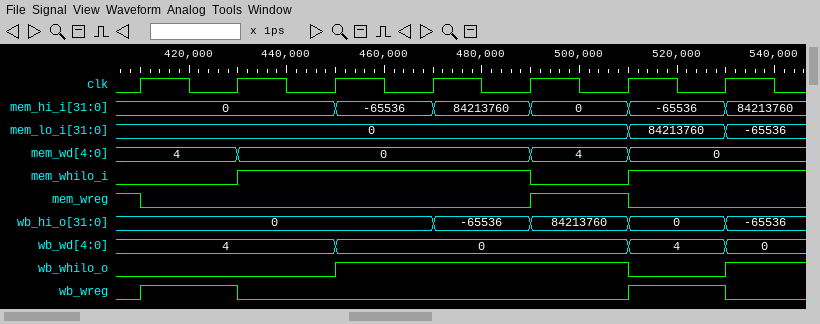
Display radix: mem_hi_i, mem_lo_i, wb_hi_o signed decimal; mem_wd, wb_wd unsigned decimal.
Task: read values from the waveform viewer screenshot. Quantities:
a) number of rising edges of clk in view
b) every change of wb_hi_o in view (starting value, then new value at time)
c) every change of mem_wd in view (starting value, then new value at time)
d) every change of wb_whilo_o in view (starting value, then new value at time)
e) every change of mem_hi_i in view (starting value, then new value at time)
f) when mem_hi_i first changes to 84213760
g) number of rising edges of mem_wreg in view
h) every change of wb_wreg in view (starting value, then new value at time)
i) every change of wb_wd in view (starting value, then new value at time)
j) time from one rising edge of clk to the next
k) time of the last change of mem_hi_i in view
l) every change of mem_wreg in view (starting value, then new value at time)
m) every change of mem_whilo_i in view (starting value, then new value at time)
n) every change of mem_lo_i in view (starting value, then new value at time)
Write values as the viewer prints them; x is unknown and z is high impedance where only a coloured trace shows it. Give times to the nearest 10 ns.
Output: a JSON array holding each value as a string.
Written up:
["7", "0, -65536 at 470 ns, 84213760 at 490 ns, 0 at 510 ns, -65536 at 530 ns", "4, 0 at 430 ns, 4 at 490 ns, 0 at 510 ns", "0, 1 at 450 ns, 0 at 510 ns, 1 at 530 ns", "0, -65536 at 450 ns, 84213760 at 470 ns, 0 at 490 ns, -65536 at 510 ns, 84213760 at 530 ns", "470 ns", "1", "0, 1 at 410 ns, 0 at 430 ns, 1 at 510 ns, 0 at 530 ns", "4, 0 at 450 ns, 4 at 510 ns, 0 at 530 ns", "20 ns", "530 ns", "1, 0 at 410 ns, 1 at 490 ns, 0 at 510 ns", "0, 1 at 430 ns, 0 at 490 ns, 1 at 510 ns", "0, 84213760 at 510 ns, -65536 at 530 ns"]
